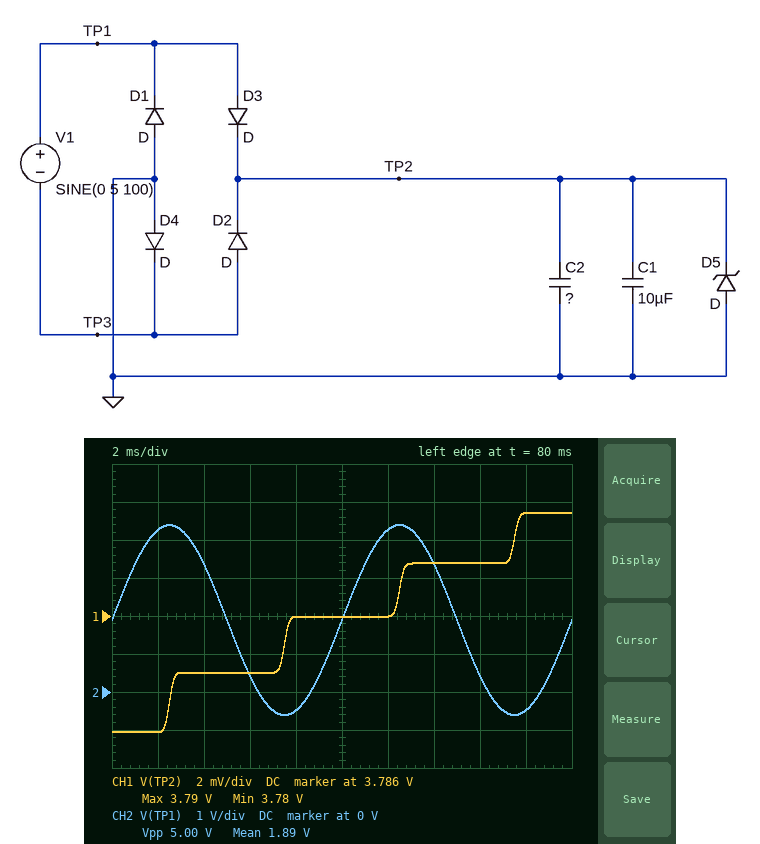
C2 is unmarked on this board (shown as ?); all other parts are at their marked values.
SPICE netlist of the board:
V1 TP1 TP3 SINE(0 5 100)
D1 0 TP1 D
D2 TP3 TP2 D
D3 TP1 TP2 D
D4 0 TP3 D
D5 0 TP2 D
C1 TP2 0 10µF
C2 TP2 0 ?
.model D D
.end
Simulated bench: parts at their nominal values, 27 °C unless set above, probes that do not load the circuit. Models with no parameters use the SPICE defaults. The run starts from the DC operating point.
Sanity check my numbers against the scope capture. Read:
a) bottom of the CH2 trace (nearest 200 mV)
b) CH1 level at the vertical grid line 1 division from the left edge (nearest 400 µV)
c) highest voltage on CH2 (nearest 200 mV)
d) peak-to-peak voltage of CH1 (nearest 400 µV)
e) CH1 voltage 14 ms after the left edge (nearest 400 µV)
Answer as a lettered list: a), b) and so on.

a) -600 mV
b) 3.7800 V
c) 4.4 V
d) 11.6 mV
e) 3.7888 V
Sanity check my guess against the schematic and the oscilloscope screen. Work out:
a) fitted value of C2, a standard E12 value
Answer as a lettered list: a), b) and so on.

a) 12 µF
